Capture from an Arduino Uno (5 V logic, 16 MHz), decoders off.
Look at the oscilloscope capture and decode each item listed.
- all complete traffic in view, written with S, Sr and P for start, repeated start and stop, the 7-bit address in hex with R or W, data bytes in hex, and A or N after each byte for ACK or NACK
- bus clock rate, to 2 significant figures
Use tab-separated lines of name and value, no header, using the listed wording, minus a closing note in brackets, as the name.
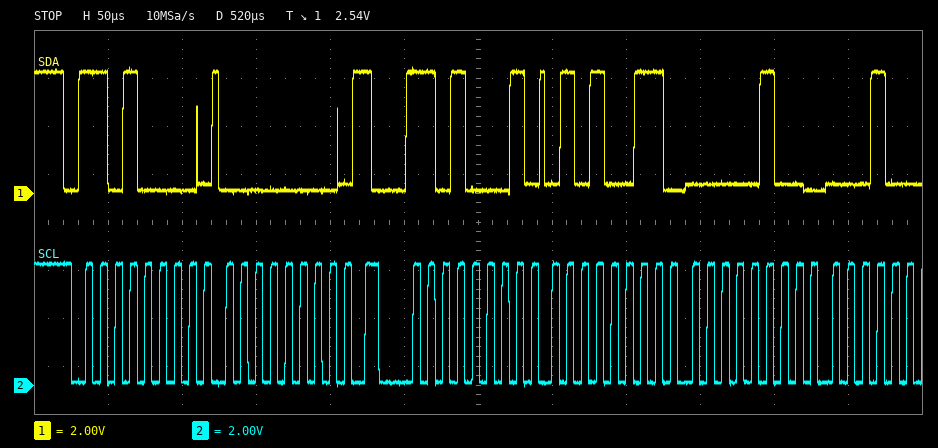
all complete traffic in view, written with S, Sr and P for start, repeated start and stop, the 7-bit address in hex with R or W, data bytes in hex, and A or N after each byte for ACK or NACK	S 68W A 00 A Sr 68R A 53 A 04 A
bus clock rate, to 2 significant figures	100 kHz
